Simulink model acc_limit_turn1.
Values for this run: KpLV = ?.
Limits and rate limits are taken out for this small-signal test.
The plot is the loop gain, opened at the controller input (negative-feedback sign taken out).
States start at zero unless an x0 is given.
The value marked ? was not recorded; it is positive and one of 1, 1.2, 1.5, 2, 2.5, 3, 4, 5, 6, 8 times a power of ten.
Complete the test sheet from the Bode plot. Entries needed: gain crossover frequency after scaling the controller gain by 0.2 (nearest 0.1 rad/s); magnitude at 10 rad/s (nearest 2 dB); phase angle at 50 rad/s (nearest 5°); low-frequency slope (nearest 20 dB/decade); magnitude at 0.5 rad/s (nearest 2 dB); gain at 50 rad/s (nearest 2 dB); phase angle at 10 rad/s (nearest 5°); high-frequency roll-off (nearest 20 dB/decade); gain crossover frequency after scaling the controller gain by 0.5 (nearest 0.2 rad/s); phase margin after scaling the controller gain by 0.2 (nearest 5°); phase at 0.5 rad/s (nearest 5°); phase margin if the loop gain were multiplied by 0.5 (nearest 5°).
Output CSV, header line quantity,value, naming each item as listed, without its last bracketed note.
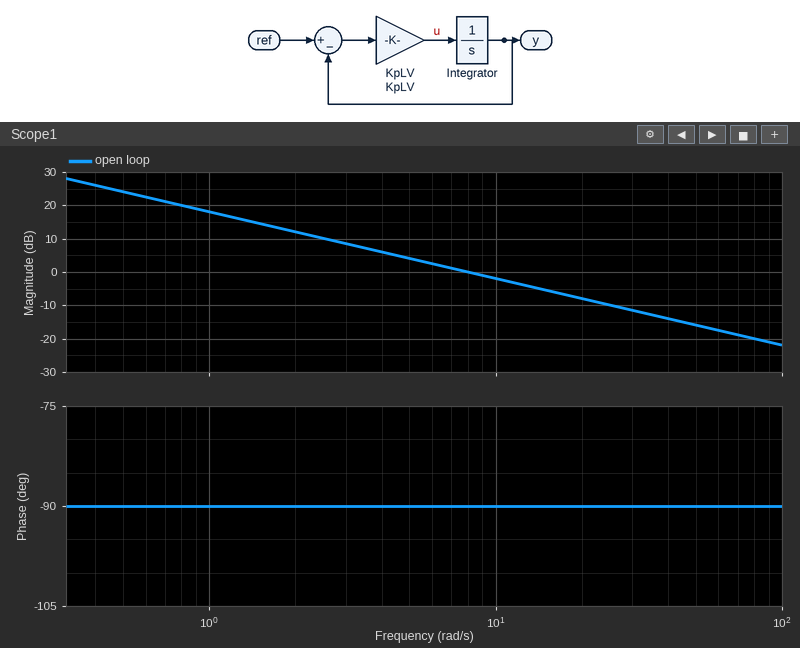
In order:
quantity,value
gain crossover frequency after scaling the controller gain by 0.2,1.6 rad/s
magnitude at 10 rad/s,-2 dB
phase angle at 50 rad/s,-90°
low-frequency slope,-20 dB/decade
magnitude at 0.5 rad/s,24 dB
gain at 50 rad/s,-16 dB
phase angle at 10 rad/s,-90°
high-frequency roll-off,-20 dB/decade
gain crossover frequency after scaling the controller gain by 0.5,4.0 rad/s
phase margin after scaling the controller gain by 0.2,90°
phase at 0.5 rad/s,-90°
phase margin if the loop gain were multiplied by 0.5,90°
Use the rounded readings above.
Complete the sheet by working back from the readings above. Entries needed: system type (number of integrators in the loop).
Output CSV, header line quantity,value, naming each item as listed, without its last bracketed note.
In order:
quantity,value
system type,1
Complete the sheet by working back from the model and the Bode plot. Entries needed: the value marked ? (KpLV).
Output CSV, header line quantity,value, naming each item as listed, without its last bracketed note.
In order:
quantity,value
the value marked ?,8
